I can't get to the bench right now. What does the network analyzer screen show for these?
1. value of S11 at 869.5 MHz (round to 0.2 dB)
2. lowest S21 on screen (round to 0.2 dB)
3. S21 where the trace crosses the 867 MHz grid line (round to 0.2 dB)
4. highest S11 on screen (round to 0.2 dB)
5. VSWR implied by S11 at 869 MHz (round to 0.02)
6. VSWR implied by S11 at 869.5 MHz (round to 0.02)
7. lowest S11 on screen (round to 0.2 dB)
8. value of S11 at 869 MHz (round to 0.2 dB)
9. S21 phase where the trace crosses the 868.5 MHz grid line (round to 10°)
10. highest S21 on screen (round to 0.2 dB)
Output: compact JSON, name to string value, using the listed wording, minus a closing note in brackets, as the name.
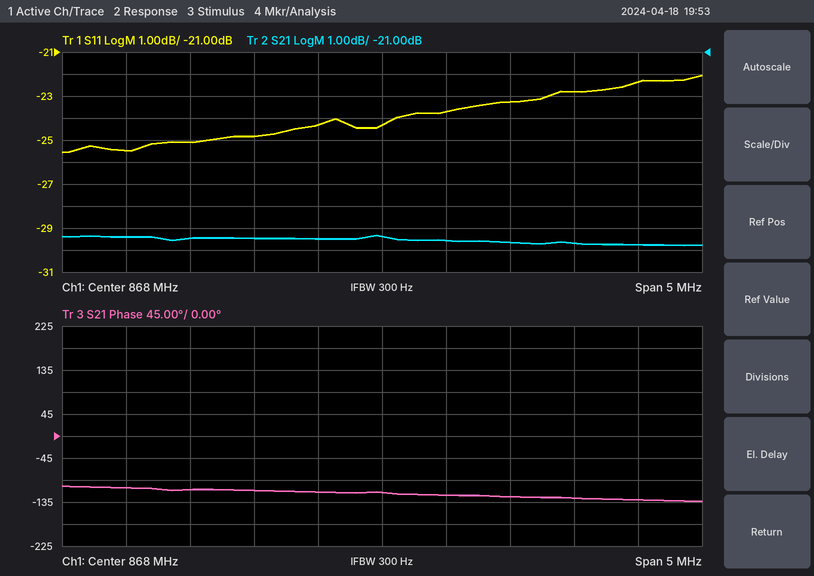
{"value of S11 at 869.5 MHz": "-22.8 dB", "lowest S21 on screen": "-29.8 dB", "S21 where the trace crosses the 867 MHz grid line": "-29.4 dB", "highest S11 on screen": "-22.0 dB", "VSWR implied by S11 at 869 MHz": "1.14", "VSWR implied by S11 at 869.5 MHz": "1.16", "lowest S11 on screen": "-25.6 dB", "value of S11 at 869 MHz": "-23.2 dB", "S21 phase where the trace crosses the 868.5 MHz grid line": "-120°", "highest S21 on screen": "-29.4 dB"}
